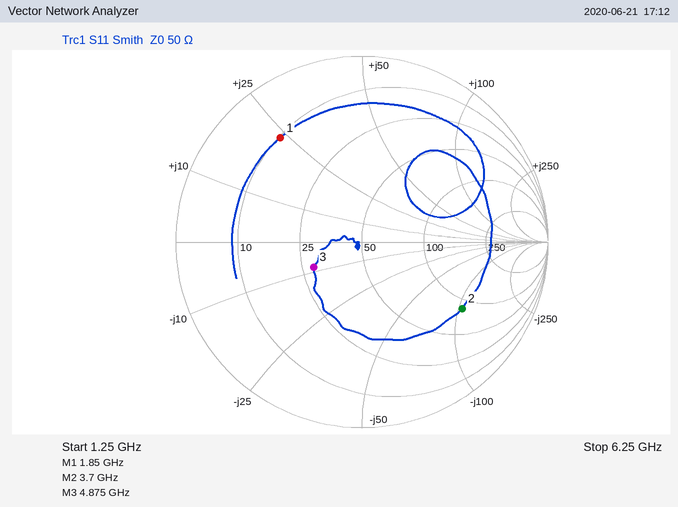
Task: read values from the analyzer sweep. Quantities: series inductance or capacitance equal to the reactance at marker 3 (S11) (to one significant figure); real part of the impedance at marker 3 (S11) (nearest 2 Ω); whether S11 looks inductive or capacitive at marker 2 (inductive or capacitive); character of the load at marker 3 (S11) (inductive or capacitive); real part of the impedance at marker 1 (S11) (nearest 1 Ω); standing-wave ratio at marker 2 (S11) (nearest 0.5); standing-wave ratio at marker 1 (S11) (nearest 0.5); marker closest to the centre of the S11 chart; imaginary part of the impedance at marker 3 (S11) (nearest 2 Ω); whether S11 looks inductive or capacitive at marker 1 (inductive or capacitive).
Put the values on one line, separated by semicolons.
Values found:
4 pF; 28 Ω; capacitive; capacitive; 10 Ω; 4.5; 6.0; marker 3; -8 Ω; inductive
